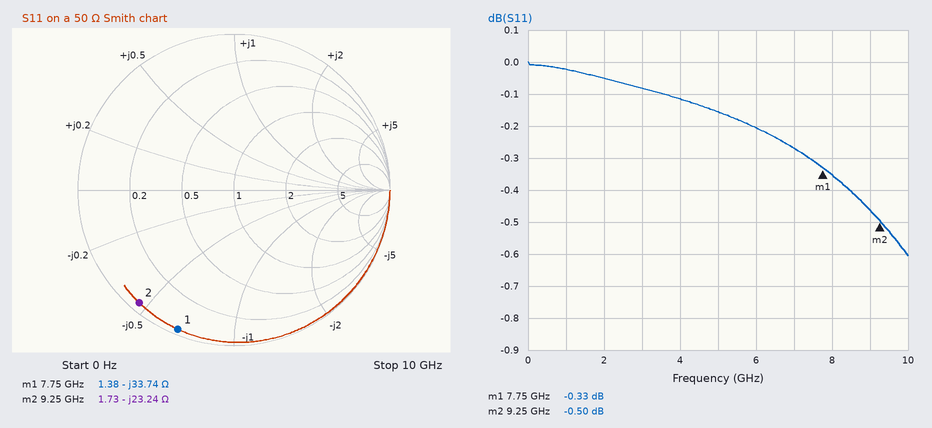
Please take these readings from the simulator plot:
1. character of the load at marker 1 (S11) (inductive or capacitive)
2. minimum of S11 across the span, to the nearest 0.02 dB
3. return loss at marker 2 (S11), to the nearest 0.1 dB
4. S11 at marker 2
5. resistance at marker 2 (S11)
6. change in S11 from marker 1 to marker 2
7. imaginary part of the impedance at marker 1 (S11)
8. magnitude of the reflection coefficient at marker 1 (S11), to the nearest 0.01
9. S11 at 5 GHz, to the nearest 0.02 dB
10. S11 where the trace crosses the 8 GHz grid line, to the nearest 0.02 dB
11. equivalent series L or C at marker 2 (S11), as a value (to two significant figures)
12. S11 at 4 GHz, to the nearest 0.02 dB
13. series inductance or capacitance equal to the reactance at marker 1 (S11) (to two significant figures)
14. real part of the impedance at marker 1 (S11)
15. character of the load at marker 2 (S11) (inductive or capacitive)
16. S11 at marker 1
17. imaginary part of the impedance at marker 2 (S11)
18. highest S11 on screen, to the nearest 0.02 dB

capacitive
-0.60 dB
0.5 dB
-0.50 dB
1.73 Ω
-0.17 dB
-33.74 Ω
0.96
-0.16 dB
-0.36 dB
740 fF
-0.12 dB
610 fF
1.38 Ω
capacitive
-0.33 dB
-23.24 Ω
0.00 dB
